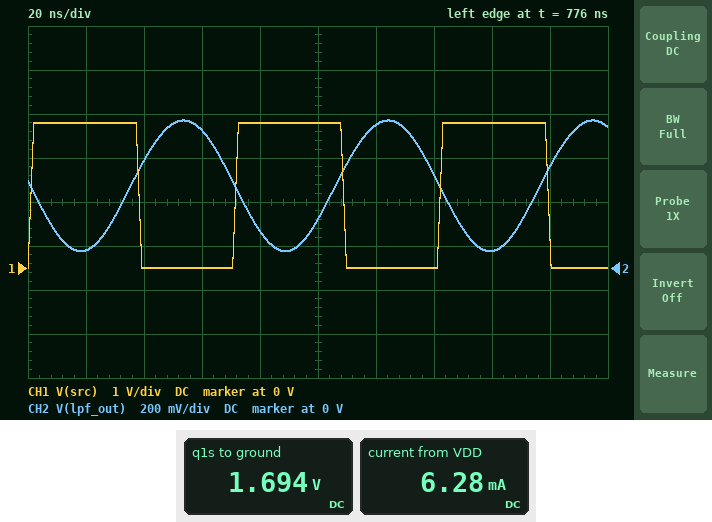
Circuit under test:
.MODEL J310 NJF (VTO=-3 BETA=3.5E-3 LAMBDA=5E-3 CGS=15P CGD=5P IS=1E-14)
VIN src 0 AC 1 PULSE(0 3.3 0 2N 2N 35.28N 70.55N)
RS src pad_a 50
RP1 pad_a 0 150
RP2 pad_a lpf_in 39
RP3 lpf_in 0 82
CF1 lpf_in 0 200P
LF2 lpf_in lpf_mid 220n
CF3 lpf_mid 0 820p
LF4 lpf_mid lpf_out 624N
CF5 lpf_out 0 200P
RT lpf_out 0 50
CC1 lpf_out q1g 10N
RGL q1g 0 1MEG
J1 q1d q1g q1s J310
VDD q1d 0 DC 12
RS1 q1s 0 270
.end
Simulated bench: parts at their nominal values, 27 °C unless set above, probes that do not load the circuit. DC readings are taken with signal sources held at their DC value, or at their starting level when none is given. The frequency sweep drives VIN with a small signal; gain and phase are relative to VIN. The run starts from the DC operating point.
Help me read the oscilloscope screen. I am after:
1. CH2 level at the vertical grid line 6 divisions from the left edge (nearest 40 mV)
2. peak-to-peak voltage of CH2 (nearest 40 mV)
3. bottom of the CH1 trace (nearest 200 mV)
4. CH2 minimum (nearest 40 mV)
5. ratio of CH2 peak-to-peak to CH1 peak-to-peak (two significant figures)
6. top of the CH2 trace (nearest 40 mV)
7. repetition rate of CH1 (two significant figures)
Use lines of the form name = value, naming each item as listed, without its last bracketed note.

CH2 level at the vertical grid line 6 divisions from the left edge = 640 mV
peak-to-peak voltage of CH2 = 600 mV
bottom of the CH1 trace = 0 V
CH2 minimum = 80 mV
ratio of CH2 peak-to-peak to CH1 peak-to-peak = 0.18
top of the CH2 trace = 680 mV
repetition rate of CH1 = 14 MHz
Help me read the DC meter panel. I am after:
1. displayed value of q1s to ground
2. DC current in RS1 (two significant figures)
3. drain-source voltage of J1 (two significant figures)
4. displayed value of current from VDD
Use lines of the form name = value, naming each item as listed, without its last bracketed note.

displayed value of q1s to ground = 1.694 V
DC current in RS1 = 6.3 mA
drain-source voltage of J1 = 10 V
displayed value of current from VDD = 6.28 mA
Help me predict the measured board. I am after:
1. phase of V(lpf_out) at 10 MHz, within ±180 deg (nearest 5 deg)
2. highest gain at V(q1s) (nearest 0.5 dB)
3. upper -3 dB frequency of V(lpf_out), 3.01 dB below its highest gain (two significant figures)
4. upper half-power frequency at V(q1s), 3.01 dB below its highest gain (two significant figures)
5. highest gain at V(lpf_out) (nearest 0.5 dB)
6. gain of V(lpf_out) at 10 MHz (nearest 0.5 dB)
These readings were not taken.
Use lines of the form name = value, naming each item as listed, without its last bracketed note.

phase of V(lpf_out) at 10 MHz, within ±180 deg = -120 deg
highest gain at V(q1s) = -16.0 dB
upper -3 dB frequency of V(lpf_out), 3.01 dB below its highest gain = 13 MHz
upper half-power frequency at V(q1s), 3.01 dB below its highest gain = 13 MHz
highest gain at V(lpf_out) = -13.5 dB
gain of V(lpf_out) at 10 MHz = -15.5 dB
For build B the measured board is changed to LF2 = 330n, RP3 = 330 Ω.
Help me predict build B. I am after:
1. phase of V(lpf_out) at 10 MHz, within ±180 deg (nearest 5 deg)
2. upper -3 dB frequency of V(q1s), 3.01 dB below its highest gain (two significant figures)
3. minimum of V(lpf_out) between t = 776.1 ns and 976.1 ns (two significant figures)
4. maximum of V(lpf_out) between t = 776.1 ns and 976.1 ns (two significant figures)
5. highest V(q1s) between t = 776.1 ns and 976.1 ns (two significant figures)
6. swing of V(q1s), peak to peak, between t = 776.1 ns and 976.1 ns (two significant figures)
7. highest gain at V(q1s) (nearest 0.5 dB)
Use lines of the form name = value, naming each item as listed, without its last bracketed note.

phase of V(lpf_out) at 10 MHz, within ±180 deg = -125 deg
upper -3 dB frequency of V(q1s), 3.01 dB below its highest gain = 11 MHz
minimum of V(lpf_out) between t = 776.1 ns and 976.1 ns = 110 mV
maximum of V(lpf_out) between t = 776.1 ns and 976.1 ns = 830 mV
highest V(q1s) between t = 776.1 ns and 976.1 ns = 2.3 V
swing of V(q1s), peak to peak, between t = 776.1 ns and 976.1 ns = 530 mV
highest gain at V(q1s) = -14.0 dB
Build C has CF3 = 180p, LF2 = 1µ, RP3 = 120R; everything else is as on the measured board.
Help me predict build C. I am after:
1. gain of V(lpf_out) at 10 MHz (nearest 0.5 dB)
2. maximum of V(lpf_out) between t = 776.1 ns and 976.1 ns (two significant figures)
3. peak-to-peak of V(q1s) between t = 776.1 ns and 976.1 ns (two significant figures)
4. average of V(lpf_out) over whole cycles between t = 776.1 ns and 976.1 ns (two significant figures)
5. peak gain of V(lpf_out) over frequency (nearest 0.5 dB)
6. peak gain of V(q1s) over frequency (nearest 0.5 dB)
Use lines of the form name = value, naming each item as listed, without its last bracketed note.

gain of V(lpf_out) at 10 MHz = -13.5 dB
maximum of V(lpf_out) between t = 776.1 ns and 976.1 ns = 760 mV
peak-to-peak of V(q1s) between t = 776.1 ns and 976.1 ns = 520 mV
average of V(lpf_out) over whole cycles between t = 776.1 ns and 976.1 ns = 410 mV
peak gain of V(lpf_out) over frequency = -12.5 dB
peak gain of V(q1s) over frequency = -15.5 dB
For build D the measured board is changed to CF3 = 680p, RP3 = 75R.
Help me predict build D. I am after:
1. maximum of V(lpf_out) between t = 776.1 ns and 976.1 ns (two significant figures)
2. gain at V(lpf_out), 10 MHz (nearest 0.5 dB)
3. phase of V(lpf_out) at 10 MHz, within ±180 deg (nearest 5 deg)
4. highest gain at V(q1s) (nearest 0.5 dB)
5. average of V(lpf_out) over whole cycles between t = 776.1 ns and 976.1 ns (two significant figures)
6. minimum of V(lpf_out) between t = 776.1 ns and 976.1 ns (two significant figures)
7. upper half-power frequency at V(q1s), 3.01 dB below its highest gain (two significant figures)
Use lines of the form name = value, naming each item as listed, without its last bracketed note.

maximum of V(lpf_out) between t = 776.1 ns and 976.1 ns = 690 mV
gain at V(lpf_out), 10 MHz = -15.0 dB
phase of V(lpf_out) at 10 MHz, within ±180 deg = -110 deg
highest gain at V(q1s) = -16.5 dB
average of V(lpf_out) over whole cycles between t = 776.1 ns and 976.1 ns = 370 mV
minimum of V(lpf_out) between t = 776.1 ns and 976.1 ns = 33 mV
upper half-power frequency at V(q1s), 3.01 dB below its highest gain = 15 MHz
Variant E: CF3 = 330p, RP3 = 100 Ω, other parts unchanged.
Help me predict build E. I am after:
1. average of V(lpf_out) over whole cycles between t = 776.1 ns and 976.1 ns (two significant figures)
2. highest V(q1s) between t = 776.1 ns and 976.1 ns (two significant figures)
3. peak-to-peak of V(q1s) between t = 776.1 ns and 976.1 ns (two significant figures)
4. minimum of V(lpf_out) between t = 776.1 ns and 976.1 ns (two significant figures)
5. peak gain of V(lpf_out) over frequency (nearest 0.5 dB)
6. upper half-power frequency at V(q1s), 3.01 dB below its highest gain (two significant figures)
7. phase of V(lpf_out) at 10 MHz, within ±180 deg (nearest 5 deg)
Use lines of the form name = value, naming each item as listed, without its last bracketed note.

average of V(lpf_out) over whole cycles between t = 776.1 ns and 976.1 ns = 400 mV
highest V(q1s) between t = 776.1 ns and 976.1 ns = 2.3 V
peak-to-peak of V(q1s) between t = 776.1 ns and 976.1 ns = 620 mV
minimum of V(lpf_out) between t = 776.1 ns and 976.1 ns = -43 mV
peak gain of V(lpf_out) over frequency = -13.0 dB
upper half-power frequency at V(q1s), 3.01 dB below its highest gain = 18 MHz
phase of V(lpf_out) at 10 MHz, within ±180 deg = -95 deg
